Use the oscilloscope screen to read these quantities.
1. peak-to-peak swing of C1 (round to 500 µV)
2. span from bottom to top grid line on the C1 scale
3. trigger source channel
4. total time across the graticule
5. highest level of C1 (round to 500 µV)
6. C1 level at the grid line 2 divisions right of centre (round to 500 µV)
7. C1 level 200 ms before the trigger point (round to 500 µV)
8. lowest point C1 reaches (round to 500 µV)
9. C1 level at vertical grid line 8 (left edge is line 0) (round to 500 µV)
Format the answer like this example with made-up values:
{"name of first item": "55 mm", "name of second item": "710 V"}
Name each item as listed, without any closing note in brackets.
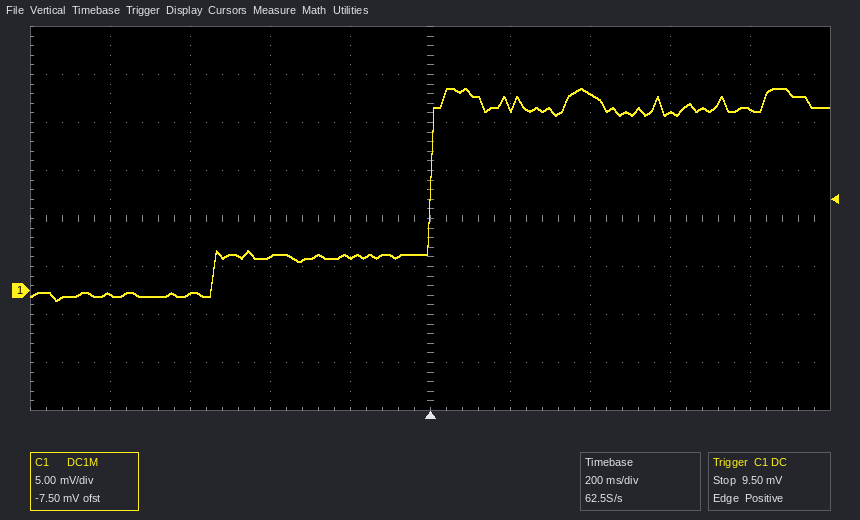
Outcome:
{"peak-to-peak swing of C1": "22.0 mV", "span from bottom to top grid line on the C1 scale": "40 mV", "trigger source channel": "C1", "total time across the graticule": "2 s", "highest level of C1": "21.0 mV", "C1 level at the grid line 2 divisions right of centre": "20.5 mV", "C1 level 200 ms before the trigger point": "3.5 mV", "lowest point C1 reaches": "-1.0 mV", "C1 level at vertical grid line 8 (left edge is line 0)": "18.5 mV"}
